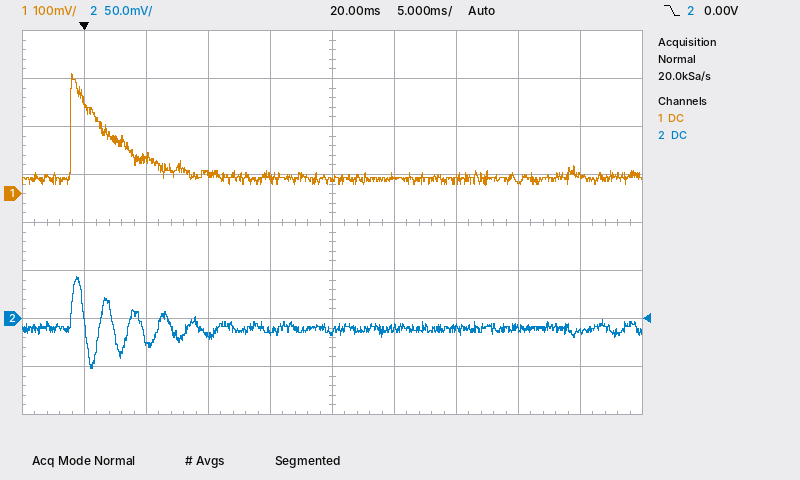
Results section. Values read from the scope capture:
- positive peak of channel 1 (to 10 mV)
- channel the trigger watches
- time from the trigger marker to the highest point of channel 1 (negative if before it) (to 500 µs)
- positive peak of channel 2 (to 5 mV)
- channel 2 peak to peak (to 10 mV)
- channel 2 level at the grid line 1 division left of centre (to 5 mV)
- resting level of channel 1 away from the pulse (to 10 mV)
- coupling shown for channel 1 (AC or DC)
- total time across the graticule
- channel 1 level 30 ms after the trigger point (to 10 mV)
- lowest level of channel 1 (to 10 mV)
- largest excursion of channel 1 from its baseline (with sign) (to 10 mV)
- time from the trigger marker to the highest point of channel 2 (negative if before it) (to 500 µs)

250 mV
channel 2
-1.0 ms
45 mV
100 mV
-15 mV
30 mV
DC
50 ms
30 mV
20 mV
+220 mV
-500 µs
